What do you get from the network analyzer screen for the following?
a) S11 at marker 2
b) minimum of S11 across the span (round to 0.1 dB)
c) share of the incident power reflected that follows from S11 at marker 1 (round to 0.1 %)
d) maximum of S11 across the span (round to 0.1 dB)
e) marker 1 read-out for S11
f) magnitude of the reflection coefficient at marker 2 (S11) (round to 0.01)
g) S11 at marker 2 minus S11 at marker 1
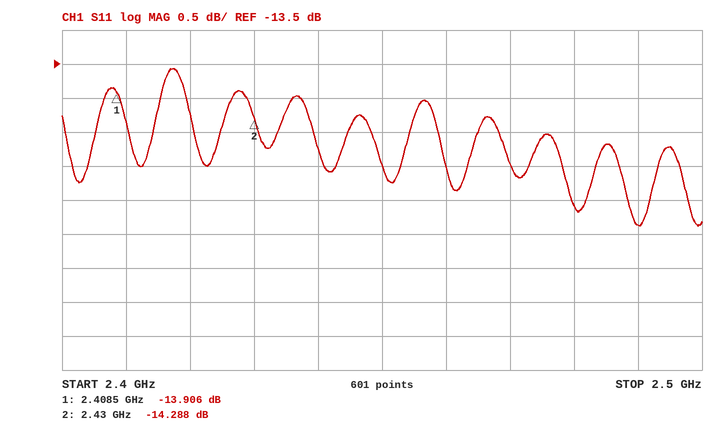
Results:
-14.288 dB
-15.9 dB
4.1 %
-13.6 dB
-13.906 dB
0.19
-0.382 dB
